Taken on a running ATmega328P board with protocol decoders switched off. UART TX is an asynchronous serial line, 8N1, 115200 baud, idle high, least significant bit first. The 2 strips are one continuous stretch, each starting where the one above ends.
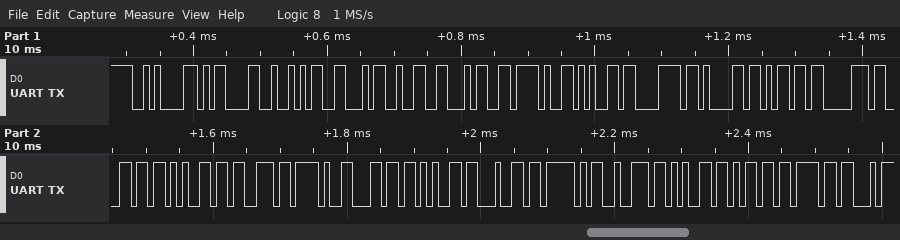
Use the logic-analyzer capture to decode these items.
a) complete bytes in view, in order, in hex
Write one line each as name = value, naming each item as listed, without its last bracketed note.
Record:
complete bytes in view, in order, in hex = 0x0A 0x0D 0x52 0x46 0x32 0x34 0x2F 0x65 0x78 0x61 0x6D 0x70 0x6C 0x65 0x73 0x2F 0x6C 0x65 0x64 0x5F 0x72 0x65 0x6D 0x6F
